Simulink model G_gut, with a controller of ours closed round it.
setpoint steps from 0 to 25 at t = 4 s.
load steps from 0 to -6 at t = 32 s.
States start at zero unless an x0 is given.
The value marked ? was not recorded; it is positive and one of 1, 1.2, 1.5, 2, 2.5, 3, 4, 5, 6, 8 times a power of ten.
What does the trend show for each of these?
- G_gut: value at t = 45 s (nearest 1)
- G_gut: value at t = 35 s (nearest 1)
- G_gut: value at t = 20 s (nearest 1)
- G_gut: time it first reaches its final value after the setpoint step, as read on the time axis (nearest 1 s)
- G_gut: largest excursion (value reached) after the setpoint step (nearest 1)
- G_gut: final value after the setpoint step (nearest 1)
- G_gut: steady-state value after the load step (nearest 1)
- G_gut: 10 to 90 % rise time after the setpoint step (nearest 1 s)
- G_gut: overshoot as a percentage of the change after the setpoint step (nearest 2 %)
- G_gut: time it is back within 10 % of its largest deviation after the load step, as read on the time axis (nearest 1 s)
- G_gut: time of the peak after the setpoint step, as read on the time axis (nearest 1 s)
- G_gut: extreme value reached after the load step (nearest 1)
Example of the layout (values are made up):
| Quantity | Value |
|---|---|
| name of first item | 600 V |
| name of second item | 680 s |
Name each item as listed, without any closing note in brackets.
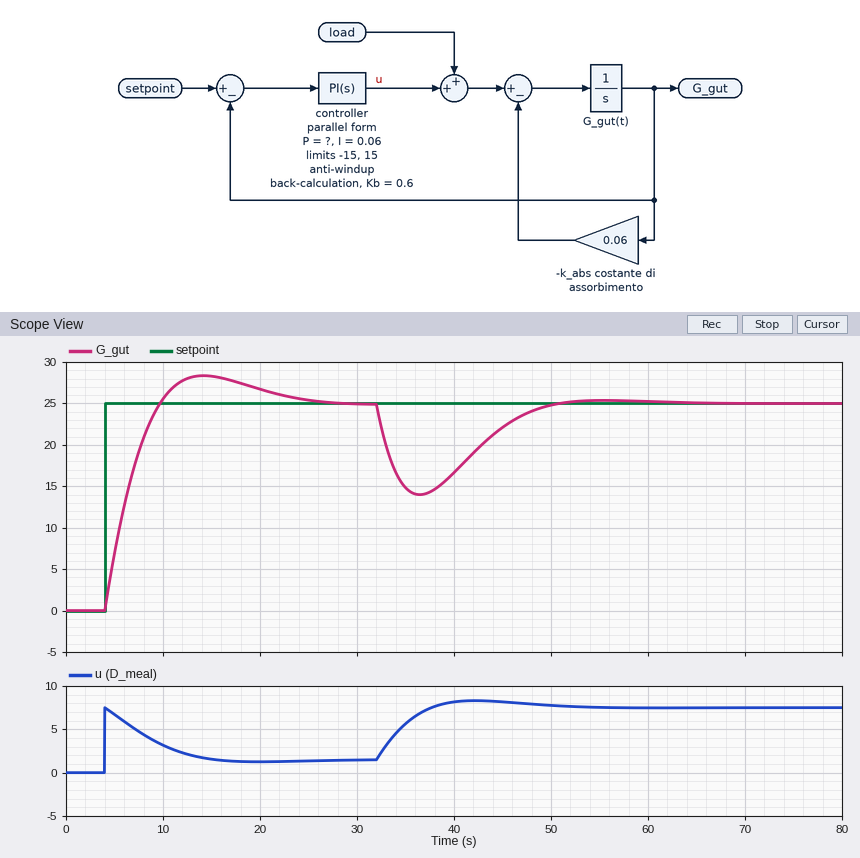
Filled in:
| Quantity | Value |
|---|---|
| G_gut: value at t = 45 s | 22 |
| G_gut: value at t = 35 s | 15 |
| G_gut: value at t = 20 s | 27 |
| G_gut: time it first reaches its final value after the setpoint step, as read on the time axis | 10 s |
| G_gut: largest excursion (value reached) after the setpoint step | 28 |
| G_gut: final value after the setpoint step | 25 |
| G_gut: steady-state value after the load step | 25 |
| G_gut: 10 to 90 % rise time after the setpoint step | 4 s |
| G_gut: overshoot as a percentage of the change after the setpoint step | 14 % |
| G_gut: time it is back within 10 % of its largest deviation after the load step, as read on the time axis | 48 s |
| G_gut: time of the peak after the setpoint step, as read on the time axis | 14 s |
| G_gut: extreme value reached after the load step | 14 |
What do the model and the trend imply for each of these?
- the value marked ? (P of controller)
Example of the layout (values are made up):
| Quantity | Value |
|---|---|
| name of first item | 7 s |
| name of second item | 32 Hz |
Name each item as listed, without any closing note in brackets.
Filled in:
| Quantity | Value |
|---|---|
| the value marked ? | 0.3 |
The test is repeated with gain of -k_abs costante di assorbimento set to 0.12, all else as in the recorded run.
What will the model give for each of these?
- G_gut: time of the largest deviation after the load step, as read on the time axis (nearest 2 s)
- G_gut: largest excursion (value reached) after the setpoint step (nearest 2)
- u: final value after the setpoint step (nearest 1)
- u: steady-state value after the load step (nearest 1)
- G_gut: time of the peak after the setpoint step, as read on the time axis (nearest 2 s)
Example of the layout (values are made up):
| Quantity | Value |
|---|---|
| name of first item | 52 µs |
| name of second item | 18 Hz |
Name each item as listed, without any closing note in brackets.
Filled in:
| Quantity | Value |
|---|---|
| G_gut: time of the largest deviation after the load step, as read on the time axis | 36 s |
| G_gut: largest excursion (value reached) after the setpoint step | 26 |
| u: final value after the setpoint step | 3 |
| u: steady-state value after the load step | 9 |
| G_gut: time of the peak after the setpoint step, as read on the time axis | 16 s |
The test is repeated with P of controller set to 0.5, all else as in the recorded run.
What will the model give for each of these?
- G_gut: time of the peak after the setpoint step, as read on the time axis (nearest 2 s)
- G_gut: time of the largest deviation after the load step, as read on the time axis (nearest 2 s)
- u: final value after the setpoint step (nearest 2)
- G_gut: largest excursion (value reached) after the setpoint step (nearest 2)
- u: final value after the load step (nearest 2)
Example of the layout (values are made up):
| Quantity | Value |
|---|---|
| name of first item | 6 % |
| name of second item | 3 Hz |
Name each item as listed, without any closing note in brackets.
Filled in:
| Quantity | Value |
|---|---|
| G_gut: time of the peak after the setpoint step, as read on the time axis | 14 s |
| G_gut: time of the largest deviation after the load step, as read on the time axis | 36 s |
| u: final value after the setpoint step | 2 |
| G_gut: largest excursion (value reached) after the setpoint step | 26 |
| u: final value after the load step | 8 |
